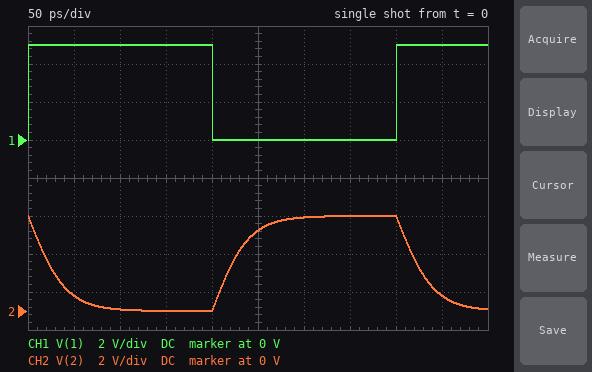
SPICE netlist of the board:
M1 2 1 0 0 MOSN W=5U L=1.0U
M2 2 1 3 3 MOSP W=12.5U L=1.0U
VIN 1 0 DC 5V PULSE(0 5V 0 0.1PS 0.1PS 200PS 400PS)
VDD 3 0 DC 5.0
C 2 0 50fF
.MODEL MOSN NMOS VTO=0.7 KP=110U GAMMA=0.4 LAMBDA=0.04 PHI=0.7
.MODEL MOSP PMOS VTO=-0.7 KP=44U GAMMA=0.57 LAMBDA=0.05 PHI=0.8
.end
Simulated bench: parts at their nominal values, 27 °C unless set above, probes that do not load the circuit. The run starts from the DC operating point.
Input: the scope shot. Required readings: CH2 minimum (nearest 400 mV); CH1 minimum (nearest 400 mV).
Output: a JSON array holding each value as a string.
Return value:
["0 V", "0 V"]
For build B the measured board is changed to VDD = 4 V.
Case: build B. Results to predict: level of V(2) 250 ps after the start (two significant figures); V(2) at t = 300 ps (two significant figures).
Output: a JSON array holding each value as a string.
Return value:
["2.9 V", "3.8 V"]
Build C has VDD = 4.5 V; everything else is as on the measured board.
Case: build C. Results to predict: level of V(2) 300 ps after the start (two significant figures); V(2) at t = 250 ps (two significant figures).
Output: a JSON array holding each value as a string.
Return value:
["4.4 V", "3.6 V"]
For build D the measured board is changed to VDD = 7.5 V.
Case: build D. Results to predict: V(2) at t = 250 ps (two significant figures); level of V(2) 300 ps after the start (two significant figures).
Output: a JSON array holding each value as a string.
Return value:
["7.3 V", "7.5 V"]
